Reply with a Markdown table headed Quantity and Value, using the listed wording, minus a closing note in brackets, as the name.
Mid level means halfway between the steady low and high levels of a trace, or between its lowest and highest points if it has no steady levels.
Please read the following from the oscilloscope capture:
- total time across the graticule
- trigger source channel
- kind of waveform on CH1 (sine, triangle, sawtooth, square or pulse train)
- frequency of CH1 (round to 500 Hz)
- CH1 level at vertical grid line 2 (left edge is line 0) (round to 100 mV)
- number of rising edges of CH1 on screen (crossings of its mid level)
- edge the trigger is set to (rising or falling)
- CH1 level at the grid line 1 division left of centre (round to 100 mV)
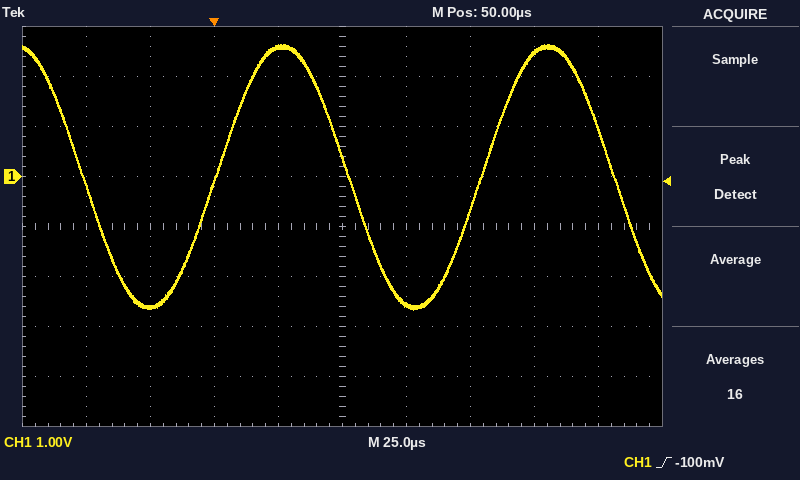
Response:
| Quantity | Value |
|---|---|
| total time across the graticule | 250 µs |
| trigger source channel | CH1 |
| kind of waveform on CH1 | sine |
| frequency of CH1 | 9.5 kHz |
| CH1 level at vertical grid line 2 (left edge is line 0) | -2.6 V |
| number of rising edges of CH1 on screen | 2 |
| edge the trigger is set to | rising |
| CH1 level at the grid line 1 division left of centre | 2.6 V |
